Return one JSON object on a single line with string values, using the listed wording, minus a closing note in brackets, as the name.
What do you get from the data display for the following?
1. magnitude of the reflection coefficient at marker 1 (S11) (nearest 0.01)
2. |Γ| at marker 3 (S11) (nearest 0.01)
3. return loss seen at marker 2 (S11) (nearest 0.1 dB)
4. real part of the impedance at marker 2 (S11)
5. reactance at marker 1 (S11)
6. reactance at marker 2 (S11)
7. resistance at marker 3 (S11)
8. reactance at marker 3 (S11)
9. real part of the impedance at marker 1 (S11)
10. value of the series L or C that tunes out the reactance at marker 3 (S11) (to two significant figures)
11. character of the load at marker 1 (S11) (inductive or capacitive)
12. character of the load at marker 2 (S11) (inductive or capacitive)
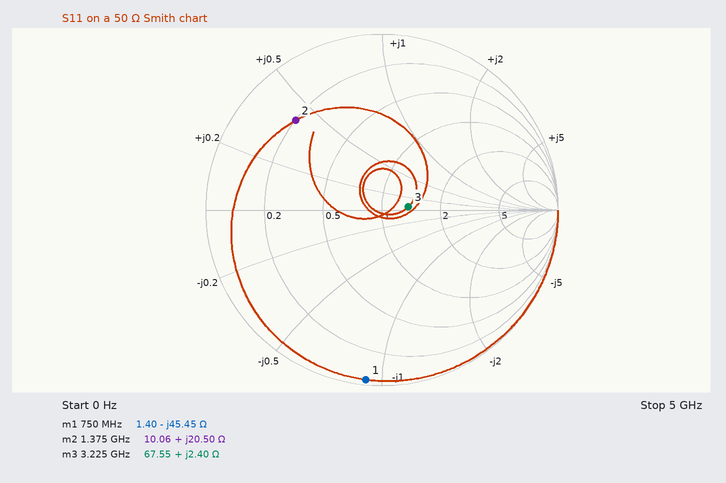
{"magnitude of the reflection coefficient at marker 1 (S11)": "0.97", "|Γ| at marker 3 (S11)": "0.15", "return loss seen at marker 2 (S11)": "3.0 dB", "real part of the impedance at marker 2": "10.06 Ω", "reactance at marker 1": "-45.45 Ω", "reactance at marker 2": "+20.50 Ω", "resistance at marker 3": "67.55 Ω", "reactance at marker 3": "+2.40 Ω", "real part of the impedance at marker 1": "1.40 Ω", "value of the series L or C that tunes out the reactance at marker 3 (S11)": "21 pF", "character of the load at marker 1 (S11)": "capacitive", "character of the load at marker 2 (S11)": "inductive"}
